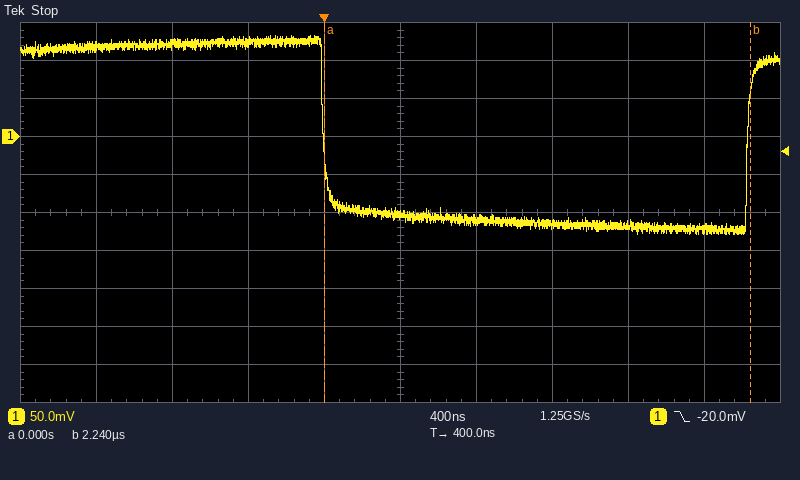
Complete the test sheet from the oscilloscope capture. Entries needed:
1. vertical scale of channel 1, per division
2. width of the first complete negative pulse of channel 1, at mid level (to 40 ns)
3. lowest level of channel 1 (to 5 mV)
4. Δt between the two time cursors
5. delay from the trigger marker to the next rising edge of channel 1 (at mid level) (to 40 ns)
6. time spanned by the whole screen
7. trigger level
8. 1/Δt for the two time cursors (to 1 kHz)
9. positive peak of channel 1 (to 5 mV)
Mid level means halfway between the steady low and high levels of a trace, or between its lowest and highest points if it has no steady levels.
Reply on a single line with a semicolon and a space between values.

50 mV; 2.24 µs; -130 mV; 2.24 µs; 2.24 µs; 4 µs; -20.0 mV; 446 kHz; 135 mV
